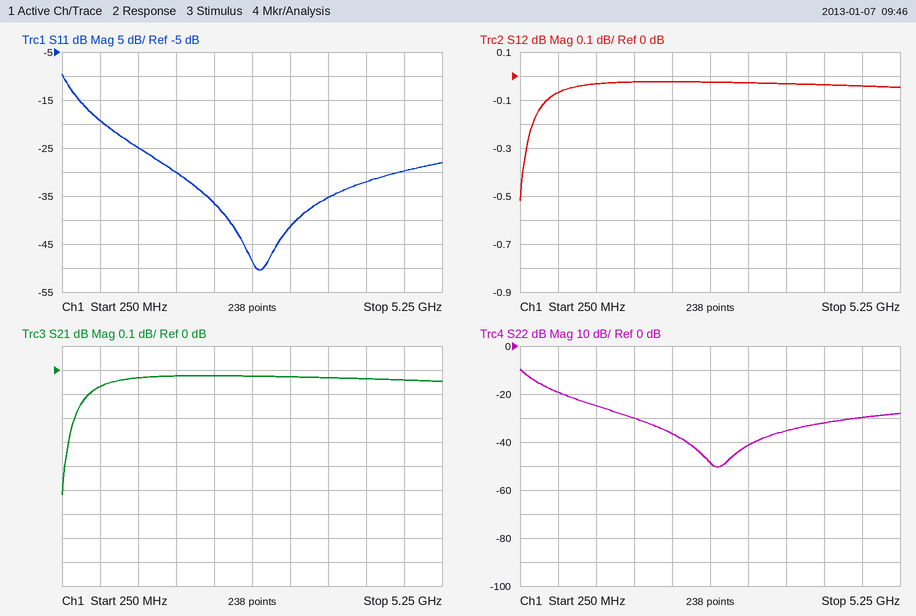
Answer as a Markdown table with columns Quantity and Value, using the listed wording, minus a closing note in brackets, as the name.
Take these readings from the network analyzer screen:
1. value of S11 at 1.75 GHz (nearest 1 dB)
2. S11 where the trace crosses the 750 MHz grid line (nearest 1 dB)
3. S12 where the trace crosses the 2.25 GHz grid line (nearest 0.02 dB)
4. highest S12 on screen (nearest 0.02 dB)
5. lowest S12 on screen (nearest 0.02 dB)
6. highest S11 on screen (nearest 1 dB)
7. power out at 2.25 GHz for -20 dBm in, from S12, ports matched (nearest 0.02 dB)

| Quantity | Value |
|---|---|
| value of S11 at 1.75 GHz | -30 dB |
| S11 where the trace crosses the 750 MHz grid line | -19 dB |
| S12 where the trace crosses the 2.25 GHz grid line | -0.02 dB |
| highest S12 on screen | -0.02 dB |
| lowest S12 on screen | -0.52 dB |
| highest S11 on screen | -10 dB |
| power out at 2.25 GHz for -20 dBm in, from S12, ports matched | -20.02 dBm |
